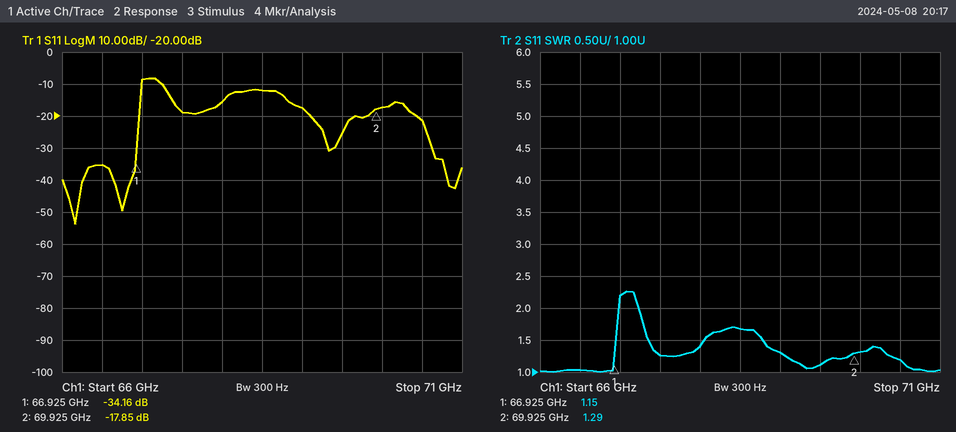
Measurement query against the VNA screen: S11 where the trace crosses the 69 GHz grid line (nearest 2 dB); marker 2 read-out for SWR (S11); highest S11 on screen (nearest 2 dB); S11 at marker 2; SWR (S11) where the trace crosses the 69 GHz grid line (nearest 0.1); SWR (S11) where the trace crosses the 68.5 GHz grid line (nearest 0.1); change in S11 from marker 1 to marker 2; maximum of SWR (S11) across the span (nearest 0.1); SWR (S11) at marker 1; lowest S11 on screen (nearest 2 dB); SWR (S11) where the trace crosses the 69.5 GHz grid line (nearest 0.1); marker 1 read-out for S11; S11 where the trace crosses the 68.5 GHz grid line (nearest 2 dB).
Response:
-18 dB
1.29
-8 dB
-17.85 dB
1.3
1.7
16.31 dB
2.3
1.15
-54 dB
1.1
-34.16 dB
-12 dB
